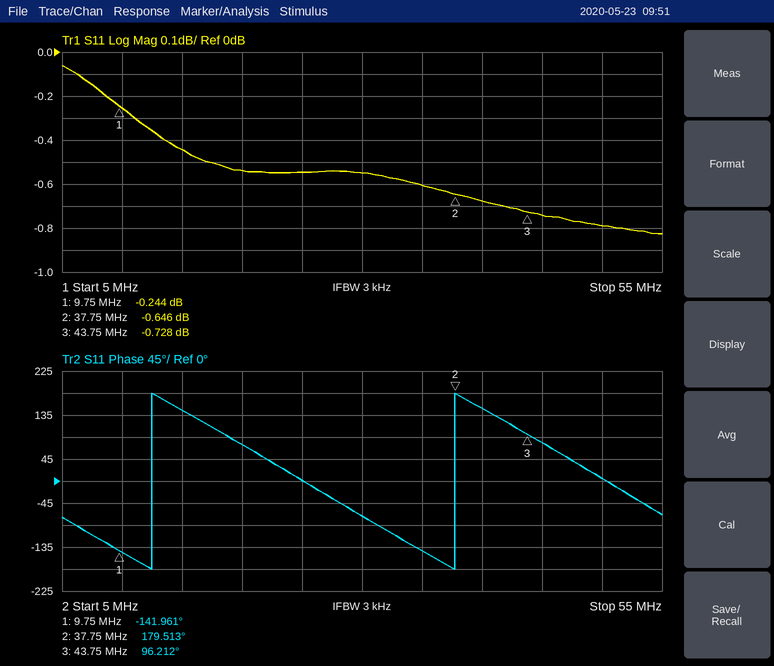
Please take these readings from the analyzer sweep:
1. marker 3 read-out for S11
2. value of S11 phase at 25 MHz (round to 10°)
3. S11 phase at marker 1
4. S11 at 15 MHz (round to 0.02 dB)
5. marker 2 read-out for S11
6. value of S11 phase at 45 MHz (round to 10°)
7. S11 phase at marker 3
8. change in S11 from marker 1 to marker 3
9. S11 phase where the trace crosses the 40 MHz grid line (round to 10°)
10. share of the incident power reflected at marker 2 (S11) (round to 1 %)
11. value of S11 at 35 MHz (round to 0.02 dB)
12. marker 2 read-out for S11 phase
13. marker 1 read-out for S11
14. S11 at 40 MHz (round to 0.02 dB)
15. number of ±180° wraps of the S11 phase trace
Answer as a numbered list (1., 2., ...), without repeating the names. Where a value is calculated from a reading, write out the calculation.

1. -0.728 dB
2. 0°
3. -141.961°
4. -0.44 dB
5. -0.646 dB
6. 80°
7. 96.212°
8. -0.728 − (-0.244) = -0.484 dB
9. 150°
10. 10^(-0.646/10) ≈ 86 %
11. -0.60 dB
12. 179.513°
13. -0.244 dB
14. -0.68 dB
15. 2
